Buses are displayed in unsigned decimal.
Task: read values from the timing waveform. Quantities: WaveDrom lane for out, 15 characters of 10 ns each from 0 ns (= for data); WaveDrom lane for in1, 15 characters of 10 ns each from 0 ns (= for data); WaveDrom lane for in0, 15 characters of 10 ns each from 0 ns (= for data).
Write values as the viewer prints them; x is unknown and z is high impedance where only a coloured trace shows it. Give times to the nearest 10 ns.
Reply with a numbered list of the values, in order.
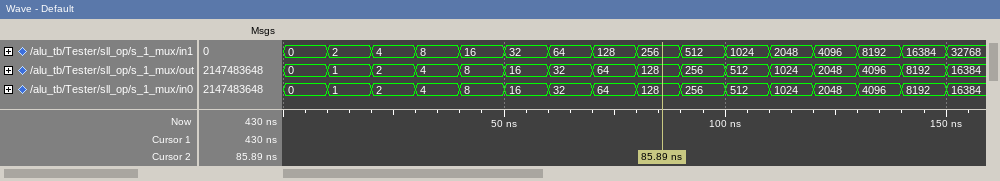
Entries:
1. {name: 'out', wave: '===============', data: '0 1 2 4 8 16 32 64 128 256 512 1024 2048 4096 8192'}
2. {name: 'in1', wave: '===============', data: '0 2 4 8 16 32 64 128 256 512 1024 2048 4096 8192 16384'}
3. {name: 'in0', wave: '===============', data: '0 1 2 4 8 16 32 64 128 256 512 1024 2048 4096 8192'}
